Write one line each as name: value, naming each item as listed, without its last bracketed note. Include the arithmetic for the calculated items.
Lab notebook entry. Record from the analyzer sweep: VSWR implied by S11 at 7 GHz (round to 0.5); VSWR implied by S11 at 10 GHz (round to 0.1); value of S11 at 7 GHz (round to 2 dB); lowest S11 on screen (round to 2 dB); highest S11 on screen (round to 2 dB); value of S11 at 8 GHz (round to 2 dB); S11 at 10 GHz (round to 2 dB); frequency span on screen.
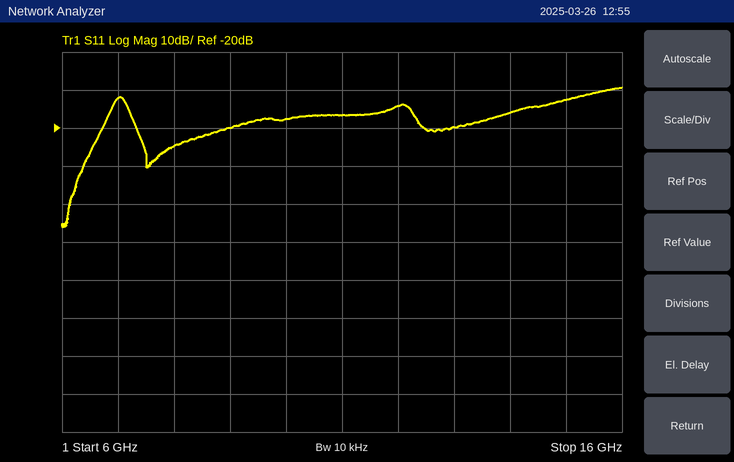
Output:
VSWR implied by S11 at 7 GHz: |Γ| = 10^(-12/20) = 0.2512; VSWR = (1 + 0.2512)/(1 − 0.2512) ≈ 1.67, so 1.5 to the nearest 0.5
VSWR implied by S11 at 10 GHz: |Γ| = 10^(-18/20) = 0.1259; VSWR = (1 + 0.1259)/(1 − 0.1259) ≈ 1.3
value of S11 at 7 GHz: -12 dB
lowest S11 on screen: -46 dB
highest S11 on screen: -10 dB
value of S11 at 8 GHz: -24 dB
S11 at 10 GHz: -18 dB
frequency span on screen: 10 GHz
